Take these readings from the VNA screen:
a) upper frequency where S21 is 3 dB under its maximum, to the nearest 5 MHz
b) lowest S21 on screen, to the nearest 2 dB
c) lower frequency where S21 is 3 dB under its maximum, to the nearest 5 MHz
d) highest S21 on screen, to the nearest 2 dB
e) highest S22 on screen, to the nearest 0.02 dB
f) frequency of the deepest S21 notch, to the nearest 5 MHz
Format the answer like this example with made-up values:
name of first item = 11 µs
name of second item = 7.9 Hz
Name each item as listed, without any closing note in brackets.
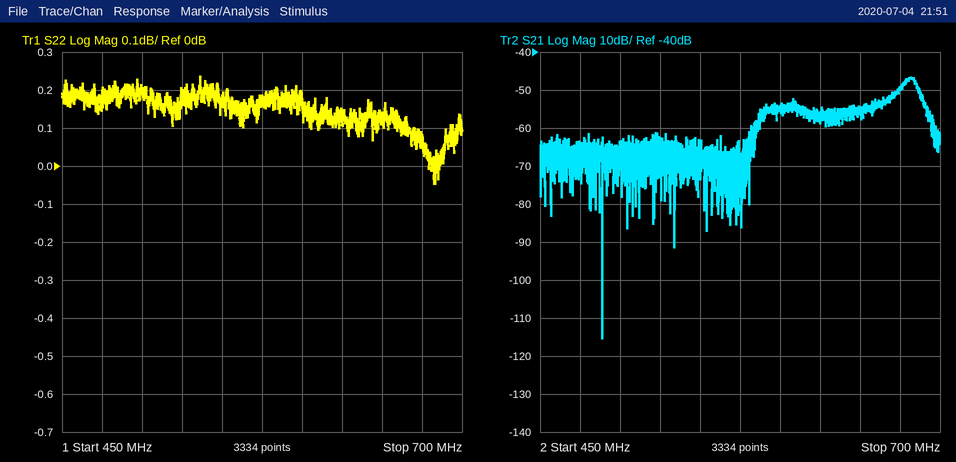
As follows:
upper frequency where S21 is 3 dB under its maximum, to the nearest 5 MHz = 685 MHz
lowest S21 on screen, to the nearest 2 dB = -116 dB
lower frequency where S21 is 3 dB under its maximum, to the nearest 5 MHz = 675 MHz
highest S21 on screen, to the nearest 2 dB = -46 dB
highest S22 on screen, to the nearest 0.02 dB = 0.24 dB
frequency of the deepest S21 notch, to the nearest 5 MHz = 490 MHz
